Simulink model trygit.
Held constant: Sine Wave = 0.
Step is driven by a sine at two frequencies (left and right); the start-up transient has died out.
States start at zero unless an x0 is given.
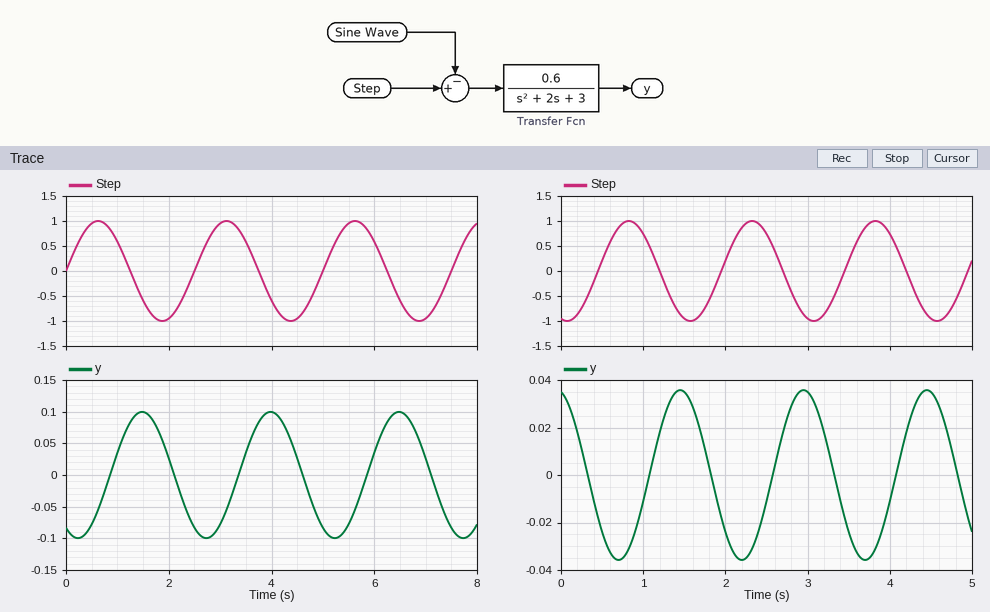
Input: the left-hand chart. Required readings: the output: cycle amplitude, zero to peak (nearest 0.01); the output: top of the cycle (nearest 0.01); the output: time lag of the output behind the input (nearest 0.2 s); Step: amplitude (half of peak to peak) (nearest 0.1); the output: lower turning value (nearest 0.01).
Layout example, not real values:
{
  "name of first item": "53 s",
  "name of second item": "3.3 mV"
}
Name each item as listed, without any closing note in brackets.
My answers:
{
  "the output: cycle amplitude, zero to peak": "0.10",
  "the output: top of the cycle": "0.10",
  "the output: time lag of the output behind the input": "0.8 s",
  "Step: amplitude (half of peak to peak)": "1.0",
  "the output: lower turning value": "-0.10"
}
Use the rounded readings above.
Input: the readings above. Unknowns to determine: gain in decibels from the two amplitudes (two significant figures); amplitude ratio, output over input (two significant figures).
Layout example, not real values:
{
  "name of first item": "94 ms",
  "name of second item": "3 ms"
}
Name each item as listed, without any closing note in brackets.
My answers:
{
  "gain in decibels from the two amplitudes": "-20 dB",
  "amplitude ratio, output over input": "0.10"
}
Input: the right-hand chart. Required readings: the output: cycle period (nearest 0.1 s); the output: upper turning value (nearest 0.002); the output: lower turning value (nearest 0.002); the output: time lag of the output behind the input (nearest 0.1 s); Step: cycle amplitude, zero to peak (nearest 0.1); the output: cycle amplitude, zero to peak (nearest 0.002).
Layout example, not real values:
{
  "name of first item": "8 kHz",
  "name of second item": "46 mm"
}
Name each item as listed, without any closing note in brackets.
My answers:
{
  "the output: cycle period": "1.5 s",
  "the output: upper turning value": "0.036",
  "the output: lower turning value": "-0.036",
  "the output: time lag of the output behind the input": "0.6 s",
  "Step: cycle amplitude, zero to peak": "1.0",
  "the output: cycle amplitude, zero to peak": "0.036"
}
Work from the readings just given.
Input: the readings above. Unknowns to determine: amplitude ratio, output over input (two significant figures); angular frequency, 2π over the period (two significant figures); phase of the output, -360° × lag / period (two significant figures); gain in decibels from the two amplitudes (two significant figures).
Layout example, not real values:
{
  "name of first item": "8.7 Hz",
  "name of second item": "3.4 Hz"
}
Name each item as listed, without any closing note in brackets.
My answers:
{
  "amplitude ratio, output over input": "0.036",
  "angular frequency, 2π over the period": "4.2 rad/s",
  "phase of the output, -360° × lag / period": "-140°",
  "gain in decibels from the two amplitudes": "-29 dB"
}
